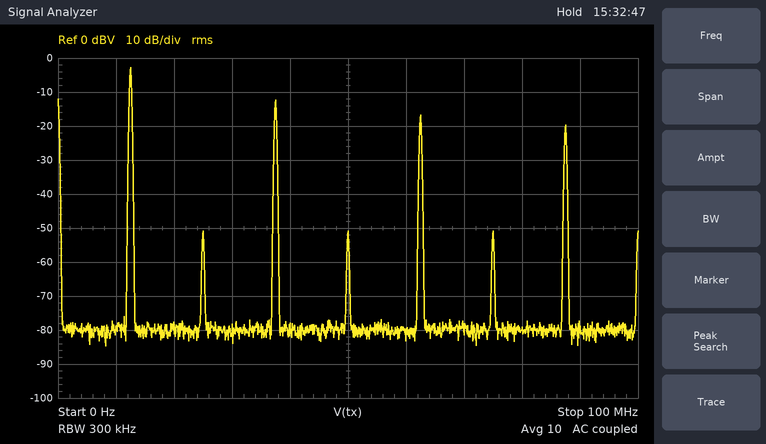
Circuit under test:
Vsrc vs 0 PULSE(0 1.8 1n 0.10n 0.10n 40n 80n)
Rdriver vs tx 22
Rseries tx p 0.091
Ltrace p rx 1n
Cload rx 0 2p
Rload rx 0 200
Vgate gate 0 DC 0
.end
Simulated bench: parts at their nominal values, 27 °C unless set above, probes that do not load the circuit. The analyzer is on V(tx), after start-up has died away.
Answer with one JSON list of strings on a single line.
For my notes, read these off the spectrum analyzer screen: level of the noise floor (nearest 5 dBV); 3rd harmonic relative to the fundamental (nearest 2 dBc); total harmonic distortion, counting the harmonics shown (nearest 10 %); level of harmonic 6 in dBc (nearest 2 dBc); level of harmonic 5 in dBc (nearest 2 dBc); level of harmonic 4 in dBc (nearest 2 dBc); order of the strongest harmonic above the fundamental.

["-80 dBV", "-10 dBc", "40 %", "-48 dBc", "-14 dBc", "-48 dBc", "3"]
